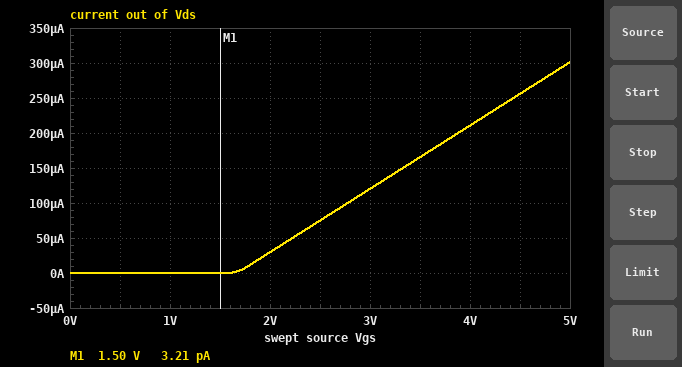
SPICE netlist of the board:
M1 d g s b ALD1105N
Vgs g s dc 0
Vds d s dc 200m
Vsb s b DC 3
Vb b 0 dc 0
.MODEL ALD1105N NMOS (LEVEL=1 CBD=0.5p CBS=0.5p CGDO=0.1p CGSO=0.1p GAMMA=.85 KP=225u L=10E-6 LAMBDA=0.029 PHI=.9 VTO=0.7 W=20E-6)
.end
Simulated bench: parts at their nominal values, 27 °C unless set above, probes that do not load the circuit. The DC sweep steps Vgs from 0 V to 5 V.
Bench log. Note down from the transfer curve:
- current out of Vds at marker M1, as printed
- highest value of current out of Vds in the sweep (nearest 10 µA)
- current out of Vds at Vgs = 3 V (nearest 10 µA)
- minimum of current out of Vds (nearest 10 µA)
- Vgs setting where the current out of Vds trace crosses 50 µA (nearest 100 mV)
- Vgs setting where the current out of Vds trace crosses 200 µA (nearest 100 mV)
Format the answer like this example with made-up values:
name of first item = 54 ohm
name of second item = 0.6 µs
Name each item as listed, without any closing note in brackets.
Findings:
current out of Vds at marker M1, as printed = 3.21 pA
highest value of current out of Vds in the sweep = 300 µA
current out of Vds at Vgs = 3 V = 120 µA
minimum of current out of Vds = 0 A
Vgs setting where the current out of Vds trace crosses 50 µA = 2.2 V
Vgs setting where the current out of Vds trace crosses 200 µA = 3.9 V
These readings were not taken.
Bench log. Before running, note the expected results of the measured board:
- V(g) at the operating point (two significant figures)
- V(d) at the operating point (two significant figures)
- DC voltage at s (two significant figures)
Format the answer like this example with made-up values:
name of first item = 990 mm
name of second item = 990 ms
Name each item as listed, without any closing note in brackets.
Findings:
V(g) at the operating point = 3.0 V
V(d) at the operating point = 3.2 V
DC voltage at s = 3.0 V
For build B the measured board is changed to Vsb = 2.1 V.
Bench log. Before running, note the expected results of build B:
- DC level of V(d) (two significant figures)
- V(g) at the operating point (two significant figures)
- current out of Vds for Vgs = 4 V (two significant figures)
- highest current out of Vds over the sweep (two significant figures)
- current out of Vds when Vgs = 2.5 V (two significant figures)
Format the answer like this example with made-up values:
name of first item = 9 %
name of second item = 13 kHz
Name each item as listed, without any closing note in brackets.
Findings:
DC level of V(d) = 2.3 V
V(g) at the operating point = 2.1 V
current out of Vds for Vgs = 4 V = 230 µA
highest current out of Vds over the sweep = 320 µA
current out of Vds when Vgs = 2.5 V = 94 µA
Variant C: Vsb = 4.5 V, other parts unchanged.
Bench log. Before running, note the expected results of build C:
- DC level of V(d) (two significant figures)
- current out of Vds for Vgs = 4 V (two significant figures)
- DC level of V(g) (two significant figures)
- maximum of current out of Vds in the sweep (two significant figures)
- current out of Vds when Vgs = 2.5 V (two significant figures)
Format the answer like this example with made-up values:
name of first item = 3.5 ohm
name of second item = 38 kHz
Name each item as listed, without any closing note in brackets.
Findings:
DC level of V(d) = 4.7 V
current out of Vds for Vgs = 4 V = 180 µA
DC level of V(g) = 4.5 V
maximum of current out of Vds in the sweep = 270 µA
current out of Vds when Vgs = 2.5 V = 48 µA
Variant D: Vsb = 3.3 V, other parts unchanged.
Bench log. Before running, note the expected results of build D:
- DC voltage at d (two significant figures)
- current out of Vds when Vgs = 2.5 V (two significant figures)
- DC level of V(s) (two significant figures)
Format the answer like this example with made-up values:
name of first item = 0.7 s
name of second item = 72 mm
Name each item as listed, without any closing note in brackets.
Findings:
DC voltage at d = 3.5 V
current out of Vds when Vgs = 2.5 V = 69 µA
DC level of V(s) = 3.3 V
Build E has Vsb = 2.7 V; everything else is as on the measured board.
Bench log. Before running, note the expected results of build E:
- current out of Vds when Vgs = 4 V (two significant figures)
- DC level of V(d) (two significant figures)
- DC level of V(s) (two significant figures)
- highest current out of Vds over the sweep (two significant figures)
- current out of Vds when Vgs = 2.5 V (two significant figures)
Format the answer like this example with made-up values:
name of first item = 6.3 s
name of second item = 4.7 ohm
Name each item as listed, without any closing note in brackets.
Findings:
current out of Vds when Vgs = 4 V = 220 µA
DC level of V(d) = 2.9 V
DC level of V(s) = 2.7 V
highest current out of Vds over the sweep = 310 µA
current out of Vds when Vgs = 2.5 V = 81 µA
